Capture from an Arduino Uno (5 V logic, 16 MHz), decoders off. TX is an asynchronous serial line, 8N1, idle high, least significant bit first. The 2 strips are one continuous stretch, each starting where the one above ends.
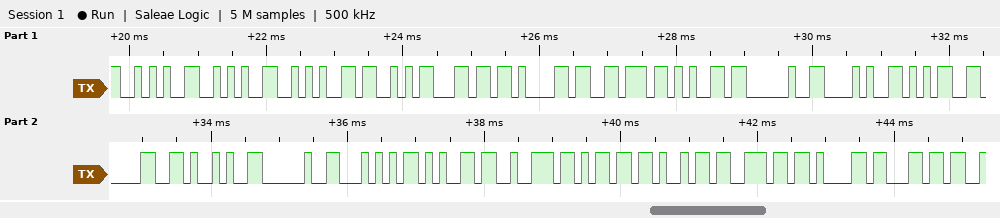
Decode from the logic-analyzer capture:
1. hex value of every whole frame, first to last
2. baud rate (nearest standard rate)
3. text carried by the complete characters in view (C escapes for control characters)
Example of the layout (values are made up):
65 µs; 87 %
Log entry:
0x2A 0x2A 0x2A 0x53 0x6C 0x61 0x76 0x65 0x20 0x28 0x35 0x30 0x29 0x20 0x54 0x65 0x72 0x6D 0x69 0x6E 0x61 0x6C; 9600 baud; "***Slave (50) Terminal"
